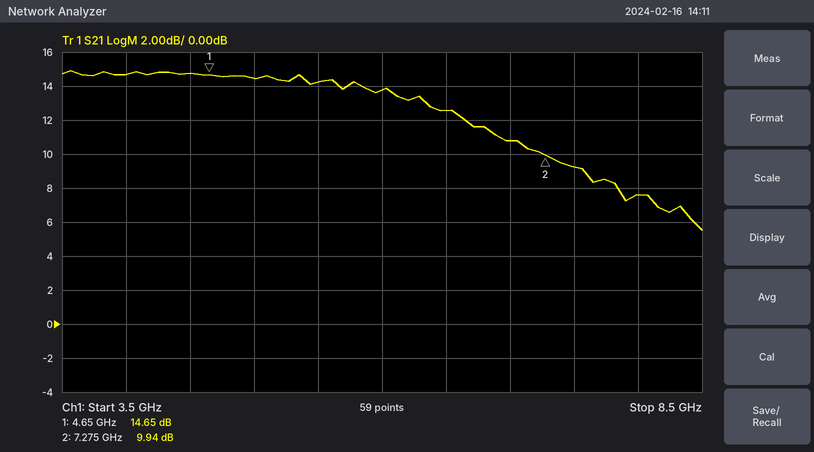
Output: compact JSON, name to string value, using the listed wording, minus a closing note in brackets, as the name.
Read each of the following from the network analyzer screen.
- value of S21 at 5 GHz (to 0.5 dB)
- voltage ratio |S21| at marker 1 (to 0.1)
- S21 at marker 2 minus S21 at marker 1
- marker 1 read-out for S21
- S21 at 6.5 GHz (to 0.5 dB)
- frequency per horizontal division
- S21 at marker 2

{"value of S21 at 5 GHz": "14.5 dB", "voltage ratio |S21| at marker 1": "5.4", "S21 at marker 2 minus S21 at marker 1": "-4.71 dB", "marker 1 read-out for S21": "14.65 dB", "S21 at 6.5 GHz": "12.5 dB", "frequency per horizontal division": "500 MHz", "S21 at marker 2": "9.94 dB"}
